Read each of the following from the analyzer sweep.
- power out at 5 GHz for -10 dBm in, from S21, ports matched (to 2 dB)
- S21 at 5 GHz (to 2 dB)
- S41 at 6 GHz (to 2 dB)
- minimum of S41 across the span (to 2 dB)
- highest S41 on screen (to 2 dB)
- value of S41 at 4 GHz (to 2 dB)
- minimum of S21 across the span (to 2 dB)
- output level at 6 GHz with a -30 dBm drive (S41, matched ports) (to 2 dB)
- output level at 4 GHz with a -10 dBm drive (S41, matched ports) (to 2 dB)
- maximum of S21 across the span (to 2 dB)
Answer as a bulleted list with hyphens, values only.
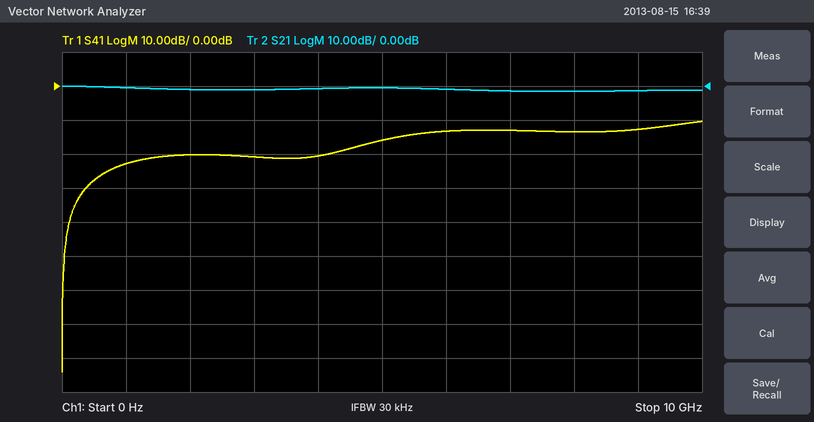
- -10 dBm
- 0 dB
- -14 dB
- -84 dB
- -10 dB
- -20 dB
- -2 dB
- -44 dBm
- -30 dBm
- 0 dB
